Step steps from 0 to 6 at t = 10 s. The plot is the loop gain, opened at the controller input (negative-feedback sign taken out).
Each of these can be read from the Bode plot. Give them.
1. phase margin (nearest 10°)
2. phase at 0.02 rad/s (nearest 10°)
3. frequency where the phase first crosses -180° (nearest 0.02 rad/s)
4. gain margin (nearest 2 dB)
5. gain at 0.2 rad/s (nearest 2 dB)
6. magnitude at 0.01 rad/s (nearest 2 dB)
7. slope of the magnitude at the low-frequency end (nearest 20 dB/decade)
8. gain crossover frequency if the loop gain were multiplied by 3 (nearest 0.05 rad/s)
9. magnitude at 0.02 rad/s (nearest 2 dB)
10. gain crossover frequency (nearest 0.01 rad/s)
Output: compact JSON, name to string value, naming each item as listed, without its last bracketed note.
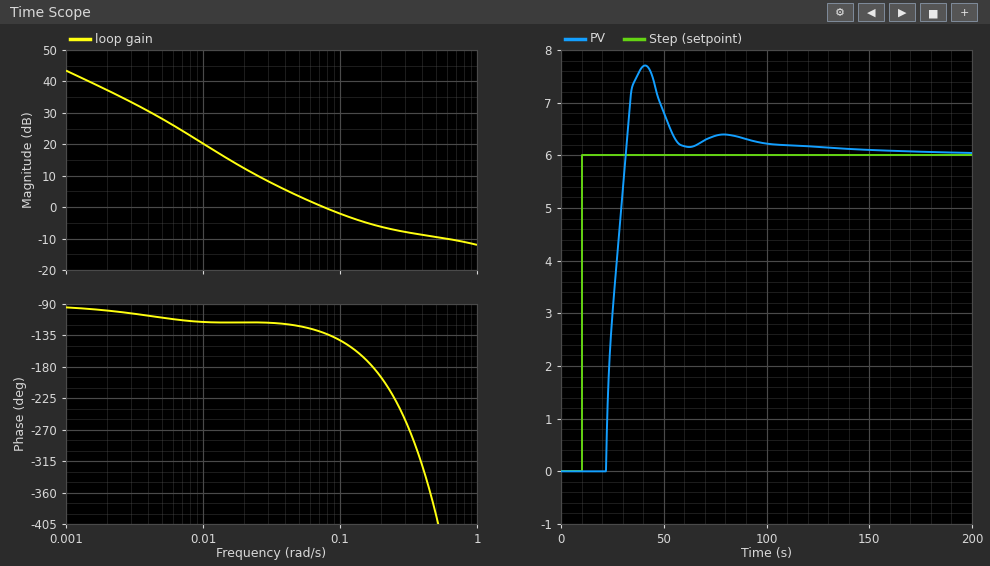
{"phase margin": "50°", "phase at 0.02 rad/s": "-120°", "frequency where the phase first crosses -180°": "0.18 rad/s", "gain margin": "6 dB", "gain at 0.2 rad/s": "-6 dB", "magnitude at 0.01 rad/s": "20 dB", "slope of the magnitude at the low-frequency end": "-20 dB/decade", "gain crossover frequency if the loop gain were multiplied by 3": "0.50 rad/s", "magnitude at 0.02 rad/s": "12 dB", "gain crossover frequency": "0.08 rad/s"}
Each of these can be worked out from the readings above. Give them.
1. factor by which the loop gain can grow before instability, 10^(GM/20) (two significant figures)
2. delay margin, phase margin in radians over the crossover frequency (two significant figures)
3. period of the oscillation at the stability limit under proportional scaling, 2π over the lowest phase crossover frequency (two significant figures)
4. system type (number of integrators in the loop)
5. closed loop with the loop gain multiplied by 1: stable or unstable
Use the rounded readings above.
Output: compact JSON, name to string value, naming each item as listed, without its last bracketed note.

{"factor by which the loop gain can grow before instability, 10^(GM/20)": "2.0", "delay margin, phase margin in radians over the crossover frequency": "11 s", "period of the oscillation at the stability limit under proportional scaling, 2π over the lowest phase crossover frequency": "35 s", "system type": "1", "closed loop with the loop gain multiplied by 1: stable or unstable": "stable"}
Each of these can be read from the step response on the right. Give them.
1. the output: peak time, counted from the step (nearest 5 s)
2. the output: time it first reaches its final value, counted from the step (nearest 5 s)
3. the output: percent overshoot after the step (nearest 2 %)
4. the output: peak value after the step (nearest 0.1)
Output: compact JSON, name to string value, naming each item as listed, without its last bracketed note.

{"the output: peak time, counted from the step": "30 s", "the output: time it first reaches its final value, counted from the step": "20 s", "the output: percent overshoot after the step": "28 %", "the output: peak value after the step": "7.7"}
